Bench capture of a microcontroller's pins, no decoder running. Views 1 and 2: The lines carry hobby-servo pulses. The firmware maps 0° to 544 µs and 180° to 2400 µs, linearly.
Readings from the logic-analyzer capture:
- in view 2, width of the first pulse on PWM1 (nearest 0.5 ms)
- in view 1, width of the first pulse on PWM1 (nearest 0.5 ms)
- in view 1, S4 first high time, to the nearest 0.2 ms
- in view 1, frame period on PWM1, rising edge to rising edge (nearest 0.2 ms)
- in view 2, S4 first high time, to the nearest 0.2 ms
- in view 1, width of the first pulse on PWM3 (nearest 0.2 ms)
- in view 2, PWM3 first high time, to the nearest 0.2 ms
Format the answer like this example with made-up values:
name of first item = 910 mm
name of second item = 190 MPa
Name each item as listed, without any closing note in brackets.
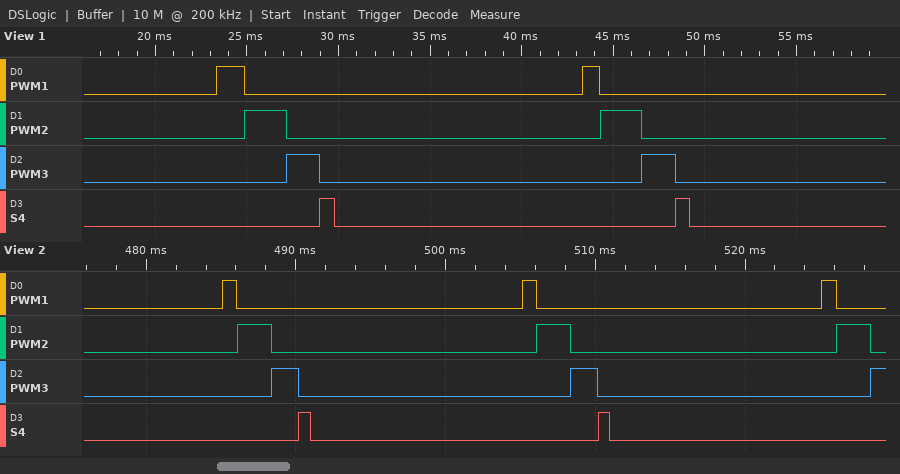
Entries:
in view 2, width of the first pulse on PWM1 = 1.0 ms
in view 1, width of the first pulse on PWM1 = 1.5 ms
in view 1, S4 first high time, to the nearest 0.2 ms = 0.8 ms
in view 1, frame period on PWM1, rising edge to rising edge = 20.0 ms
in view 2, S4 first high time, to the nearest 0.2 ms = 0.8 ms
in view 1, width of the first pulse on PWM3 = 1.8 ms
in view 2, PWM3 first high time, to the nearest 0.2 ms = 1.8 ms
